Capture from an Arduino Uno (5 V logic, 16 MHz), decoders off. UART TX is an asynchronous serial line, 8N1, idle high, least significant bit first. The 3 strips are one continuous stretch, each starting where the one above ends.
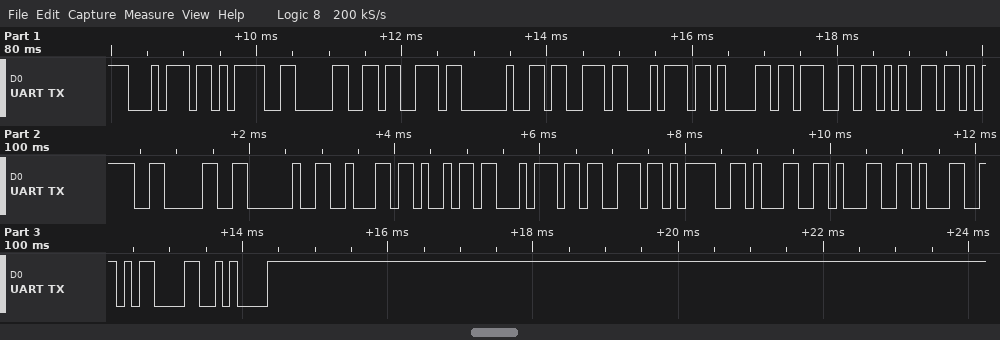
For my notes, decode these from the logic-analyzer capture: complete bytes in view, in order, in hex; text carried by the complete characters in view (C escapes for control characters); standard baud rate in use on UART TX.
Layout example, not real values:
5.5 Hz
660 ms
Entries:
0x74 0x3D 0x30 0x73 0x20 0x73 0x74 0x61 0x67 0x65 0x3D 0x30 0x20 0x62 0x69 0x74 0x73 0x3D 0x31 0x31 0x31 0x0D 0x0A
"t=0s stage=0 bits=111\r\n"
9600 baud
